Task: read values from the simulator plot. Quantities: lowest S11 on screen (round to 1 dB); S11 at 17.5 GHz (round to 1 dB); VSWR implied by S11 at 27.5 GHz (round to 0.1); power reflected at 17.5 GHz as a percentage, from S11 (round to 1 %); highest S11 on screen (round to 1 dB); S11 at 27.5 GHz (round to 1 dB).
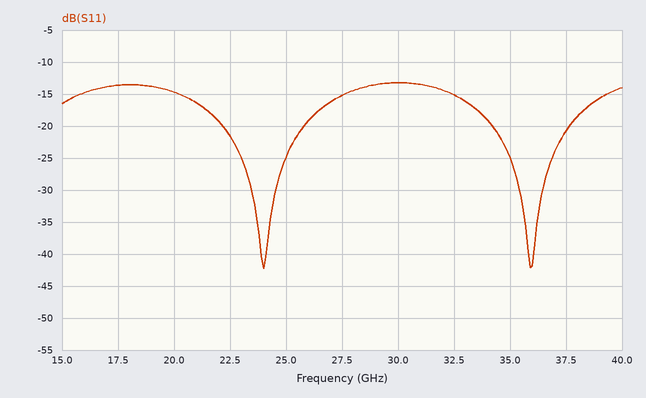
-42 dB
-14 dB
1.4
4 %
-13 dB
-15 dB
